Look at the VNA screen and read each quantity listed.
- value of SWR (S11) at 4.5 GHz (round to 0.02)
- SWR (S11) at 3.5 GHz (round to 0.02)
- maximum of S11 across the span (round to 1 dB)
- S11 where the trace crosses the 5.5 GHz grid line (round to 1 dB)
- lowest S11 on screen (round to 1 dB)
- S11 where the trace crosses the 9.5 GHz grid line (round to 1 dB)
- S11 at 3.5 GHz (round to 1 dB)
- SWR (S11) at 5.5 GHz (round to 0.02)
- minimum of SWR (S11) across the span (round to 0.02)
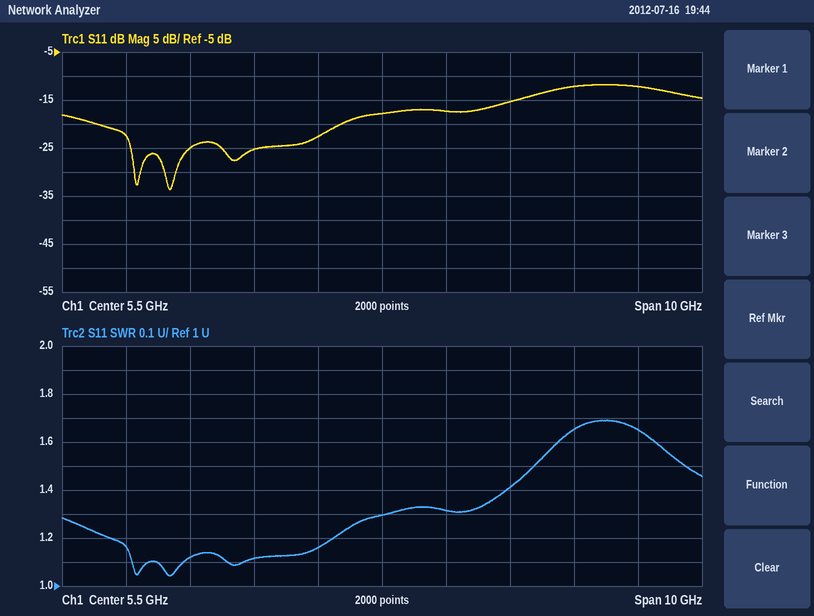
1.16
1.12
-12 dB
-18 dB
-34 dB
-12 dB
-25 dB
1.30
1.04
